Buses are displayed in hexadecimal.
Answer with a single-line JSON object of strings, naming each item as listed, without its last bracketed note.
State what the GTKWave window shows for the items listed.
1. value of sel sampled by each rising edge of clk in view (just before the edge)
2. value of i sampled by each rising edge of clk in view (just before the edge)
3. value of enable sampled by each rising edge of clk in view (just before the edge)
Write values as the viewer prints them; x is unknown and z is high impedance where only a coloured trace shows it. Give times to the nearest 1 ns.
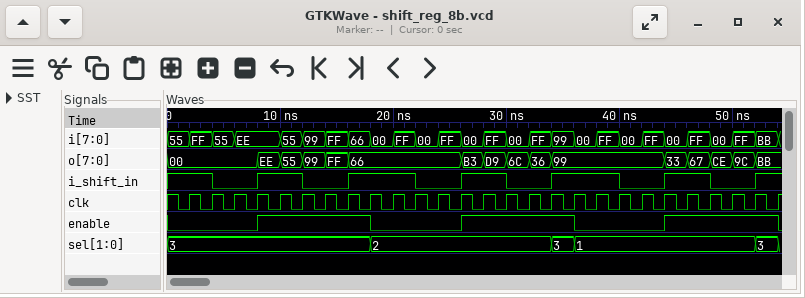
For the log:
{"value of sel sampled by each rising edge of clk in view": "3, 3, 3, 3, 3, 3, 3, 3, 3, 2, 2, 2, 2, 2, 2, 2, 2, 3, 1, 1, 1, 1, 1, 1, 1, 1, 3", "value of i sampled by each rising edge of clk in view": "55, FF, 55, EE, EE, 55, 99, FF, 66, 00, FF, 00, FF, 00, FF, 00, FF, 99, 00, FF, 00, FF, 00, FF, 00, FF, BB", "value of enable sampled by each rising edge of clk in view": "0 0 0 0 1 1 1 1 1 0 0 0 0 1 1 1 1 1 0 0 0 0 1 1 1 1 1"}
